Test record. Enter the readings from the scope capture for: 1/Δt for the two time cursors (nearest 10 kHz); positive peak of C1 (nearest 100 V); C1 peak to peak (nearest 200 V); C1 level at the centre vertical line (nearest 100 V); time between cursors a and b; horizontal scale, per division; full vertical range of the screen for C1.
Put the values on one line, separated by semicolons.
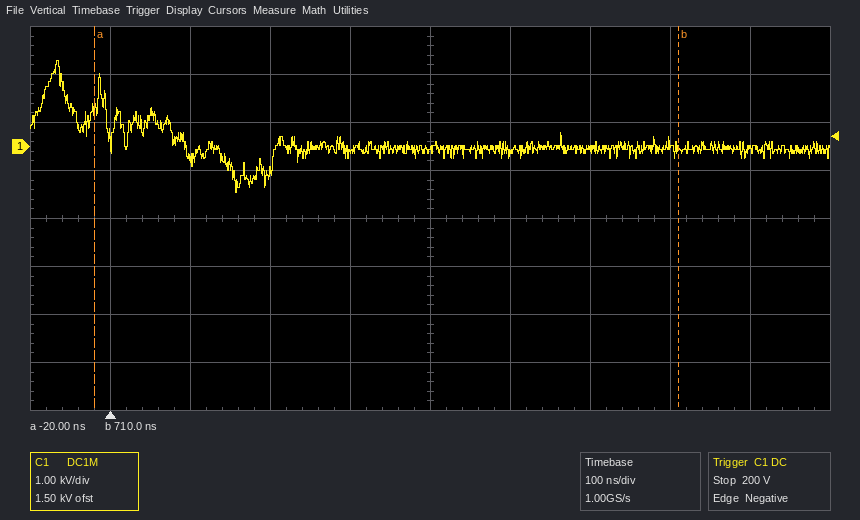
1.37 MHz; 1.8 kV; 2.8 kV; -100 V; 730 ns; 100 ns; 8 kV
